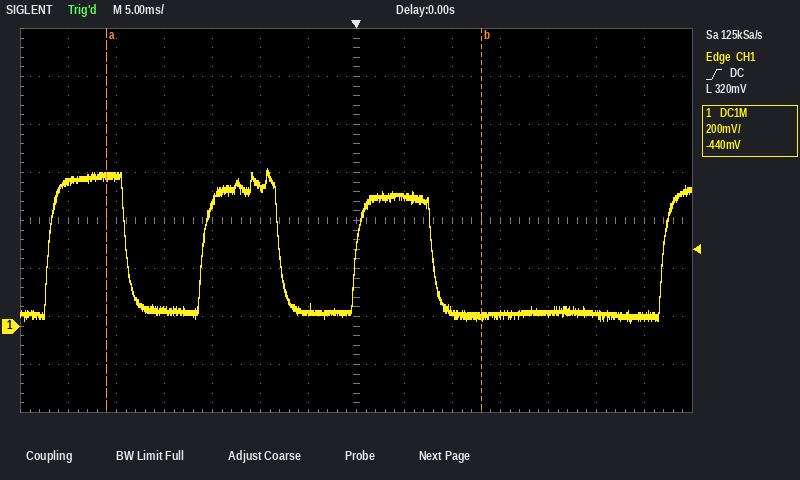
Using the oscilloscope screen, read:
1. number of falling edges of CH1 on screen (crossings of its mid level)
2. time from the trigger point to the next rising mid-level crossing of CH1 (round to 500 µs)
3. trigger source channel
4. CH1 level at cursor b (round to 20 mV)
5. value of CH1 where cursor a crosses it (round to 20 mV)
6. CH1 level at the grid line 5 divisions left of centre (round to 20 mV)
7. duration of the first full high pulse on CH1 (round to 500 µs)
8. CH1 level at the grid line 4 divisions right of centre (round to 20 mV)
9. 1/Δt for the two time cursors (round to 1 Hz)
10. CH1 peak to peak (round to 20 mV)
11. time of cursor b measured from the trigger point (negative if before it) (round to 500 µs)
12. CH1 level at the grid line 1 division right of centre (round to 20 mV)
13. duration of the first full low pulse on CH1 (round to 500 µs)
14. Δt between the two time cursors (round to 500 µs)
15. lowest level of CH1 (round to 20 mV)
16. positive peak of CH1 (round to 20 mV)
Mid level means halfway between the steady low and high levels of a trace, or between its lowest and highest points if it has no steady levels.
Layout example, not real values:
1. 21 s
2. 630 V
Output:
1. 3
2. 32.0 ms
3. CH1
4. 40 mV
5. 620 mV
6. 620 mV
7. 8.0 ms
8. 60 mV
9. 26 Hz
10. 640 mV
11. +13.0 ms
12. 540 mV
13. 8.0 ms
14. 39.0 ms
15. 20 mV
16. 660 mV
